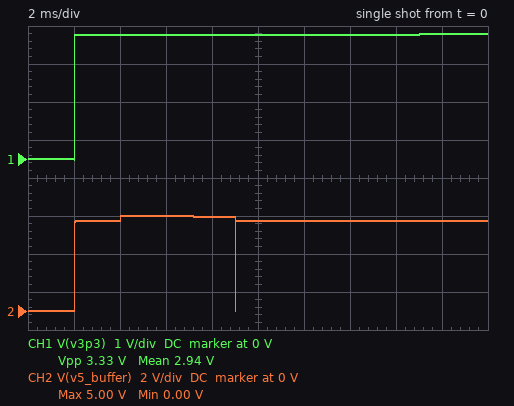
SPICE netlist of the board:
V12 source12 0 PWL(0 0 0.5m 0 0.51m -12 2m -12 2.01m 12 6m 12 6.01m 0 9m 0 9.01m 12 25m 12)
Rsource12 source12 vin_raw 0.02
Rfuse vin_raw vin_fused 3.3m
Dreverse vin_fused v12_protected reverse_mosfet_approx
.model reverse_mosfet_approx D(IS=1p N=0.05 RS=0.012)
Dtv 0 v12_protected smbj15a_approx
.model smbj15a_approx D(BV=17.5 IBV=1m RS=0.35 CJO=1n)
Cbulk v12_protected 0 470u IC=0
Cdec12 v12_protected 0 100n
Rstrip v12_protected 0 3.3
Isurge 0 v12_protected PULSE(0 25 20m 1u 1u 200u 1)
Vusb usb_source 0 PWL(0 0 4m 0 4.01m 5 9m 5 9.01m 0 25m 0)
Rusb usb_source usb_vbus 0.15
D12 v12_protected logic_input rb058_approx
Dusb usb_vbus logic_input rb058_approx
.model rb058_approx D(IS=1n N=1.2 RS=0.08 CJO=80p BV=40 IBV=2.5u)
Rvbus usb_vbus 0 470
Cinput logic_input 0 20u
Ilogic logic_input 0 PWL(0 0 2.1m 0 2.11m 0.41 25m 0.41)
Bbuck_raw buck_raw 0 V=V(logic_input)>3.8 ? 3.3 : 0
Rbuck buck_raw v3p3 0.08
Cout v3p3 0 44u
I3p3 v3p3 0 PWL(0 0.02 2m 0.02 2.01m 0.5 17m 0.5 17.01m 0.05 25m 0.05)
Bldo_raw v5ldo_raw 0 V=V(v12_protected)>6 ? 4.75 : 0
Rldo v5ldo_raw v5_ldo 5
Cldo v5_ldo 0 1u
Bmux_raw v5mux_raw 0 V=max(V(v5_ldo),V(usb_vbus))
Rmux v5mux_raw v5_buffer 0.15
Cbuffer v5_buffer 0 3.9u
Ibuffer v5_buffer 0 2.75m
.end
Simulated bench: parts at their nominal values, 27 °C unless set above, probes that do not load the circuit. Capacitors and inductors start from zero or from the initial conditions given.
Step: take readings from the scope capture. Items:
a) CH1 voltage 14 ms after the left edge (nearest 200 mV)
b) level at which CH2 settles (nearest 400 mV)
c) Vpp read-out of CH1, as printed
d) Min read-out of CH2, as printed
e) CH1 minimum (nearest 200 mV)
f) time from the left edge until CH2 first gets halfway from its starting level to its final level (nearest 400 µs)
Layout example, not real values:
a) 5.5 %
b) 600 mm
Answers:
a) 3.2 V
b) 4.8 V
c) 3.33 V
d) 0.00 V
e) 0 V
f) 2.0 ms
